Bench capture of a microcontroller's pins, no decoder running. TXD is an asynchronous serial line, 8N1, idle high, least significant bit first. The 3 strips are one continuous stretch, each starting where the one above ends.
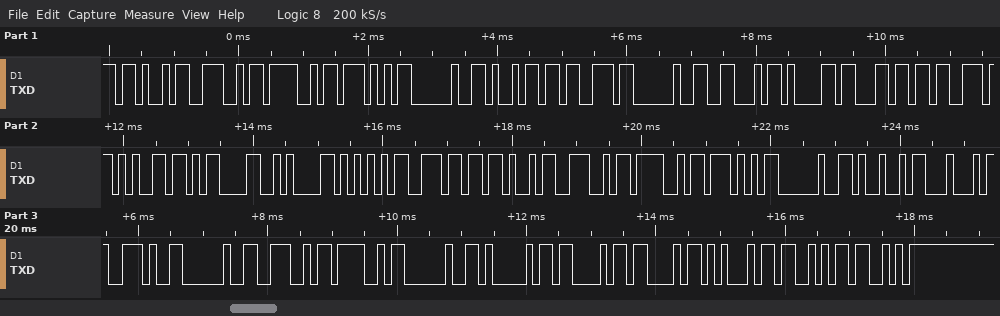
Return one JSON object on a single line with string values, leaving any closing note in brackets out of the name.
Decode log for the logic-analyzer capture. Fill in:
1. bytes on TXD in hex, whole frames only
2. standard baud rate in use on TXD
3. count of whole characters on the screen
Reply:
{"bytes on TXD in hex, whole frames only": "4B 4E 4F 57 20 69 73 20 46 61 6C 73 65 0D 0A 55 6E 4B 4E 4F 57 20 49 44 2E 20 4E 4F 20 41 43 43 45 53 53", "standard baud rate in use on TXD": "9600 baud", "count of whole characters on the screen": "35"}
